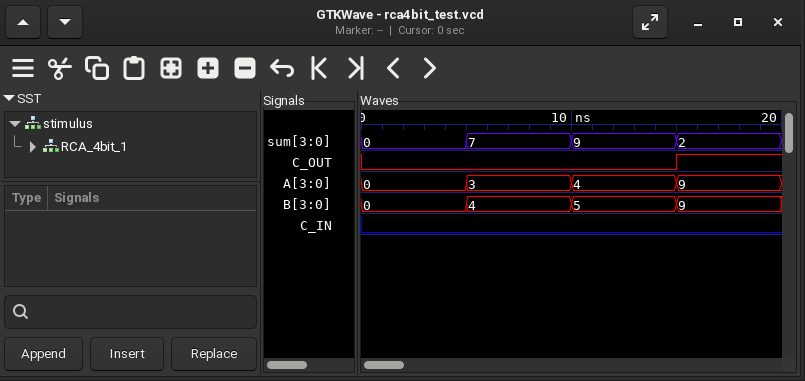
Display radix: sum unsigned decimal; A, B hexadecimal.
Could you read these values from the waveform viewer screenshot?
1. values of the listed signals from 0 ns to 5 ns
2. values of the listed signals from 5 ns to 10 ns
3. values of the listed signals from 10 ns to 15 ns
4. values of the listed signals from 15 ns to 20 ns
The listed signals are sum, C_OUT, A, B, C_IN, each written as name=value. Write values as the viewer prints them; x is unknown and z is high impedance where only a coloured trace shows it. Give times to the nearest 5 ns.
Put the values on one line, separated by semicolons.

sum=0, C_OUT=0, A=0, B=0, C_IN=0; sum=7, C_OUT=0, A=3, B=4, C_IN=0; sum=9, C_OUT=0, A=4, B=5, C_IN=0; sum=2, C_OUT=1, A=9, B=9, C_IN=0
